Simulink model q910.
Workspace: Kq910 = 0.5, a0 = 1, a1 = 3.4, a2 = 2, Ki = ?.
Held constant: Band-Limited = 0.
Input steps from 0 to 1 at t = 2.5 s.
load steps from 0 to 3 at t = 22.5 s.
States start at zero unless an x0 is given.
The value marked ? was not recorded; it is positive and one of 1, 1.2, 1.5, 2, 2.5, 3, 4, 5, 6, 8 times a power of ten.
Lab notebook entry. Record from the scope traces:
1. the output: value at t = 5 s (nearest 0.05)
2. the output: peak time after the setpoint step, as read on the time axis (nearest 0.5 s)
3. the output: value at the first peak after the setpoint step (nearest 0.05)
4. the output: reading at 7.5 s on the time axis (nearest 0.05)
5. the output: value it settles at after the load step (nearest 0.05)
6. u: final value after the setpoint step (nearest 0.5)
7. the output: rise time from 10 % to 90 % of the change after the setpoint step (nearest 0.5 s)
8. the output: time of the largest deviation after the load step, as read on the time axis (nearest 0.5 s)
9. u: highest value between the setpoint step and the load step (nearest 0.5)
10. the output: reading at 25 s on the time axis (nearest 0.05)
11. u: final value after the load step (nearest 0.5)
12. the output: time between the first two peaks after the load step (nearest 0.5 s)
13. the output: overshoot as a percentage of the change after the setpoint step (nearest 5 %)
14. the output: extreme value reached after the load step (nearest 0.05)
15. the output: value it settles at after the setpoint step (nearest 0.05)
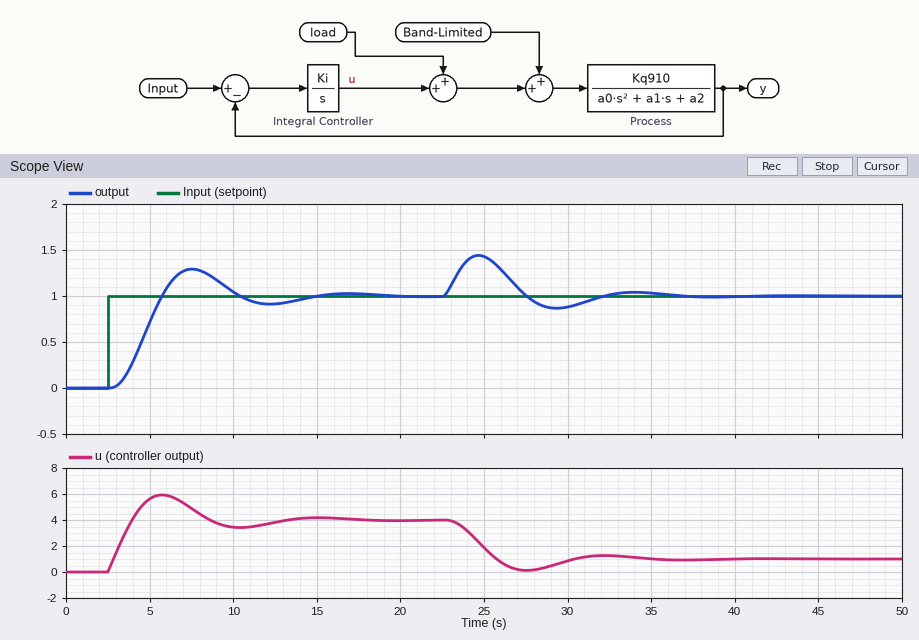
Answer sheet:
0.70
7.5 s
1.30
1.30
1.00
4.0
2.0 s
24.5 s
6.0
1.45
1.0
9.5 s
30 %
1.45
1.00
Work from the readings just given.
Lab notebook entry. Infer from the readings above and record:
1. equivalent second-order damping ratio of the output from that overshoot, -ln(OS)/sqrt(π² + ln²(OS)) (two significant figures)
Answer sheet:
0.36
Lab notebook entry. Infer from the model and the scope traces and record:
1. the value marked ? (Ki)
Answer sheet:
3
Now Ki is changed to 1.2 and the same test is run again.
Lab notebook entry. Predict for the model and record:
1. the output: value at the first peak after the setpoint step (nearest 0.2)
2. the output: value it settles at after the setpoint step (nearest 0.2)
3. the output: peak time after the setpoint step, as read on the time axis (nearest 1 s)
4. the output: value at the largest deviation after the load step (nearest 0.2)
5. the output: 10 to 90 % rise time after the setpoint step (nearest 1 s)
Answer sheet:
1.0
1.0
12 s
1.6
5 s
